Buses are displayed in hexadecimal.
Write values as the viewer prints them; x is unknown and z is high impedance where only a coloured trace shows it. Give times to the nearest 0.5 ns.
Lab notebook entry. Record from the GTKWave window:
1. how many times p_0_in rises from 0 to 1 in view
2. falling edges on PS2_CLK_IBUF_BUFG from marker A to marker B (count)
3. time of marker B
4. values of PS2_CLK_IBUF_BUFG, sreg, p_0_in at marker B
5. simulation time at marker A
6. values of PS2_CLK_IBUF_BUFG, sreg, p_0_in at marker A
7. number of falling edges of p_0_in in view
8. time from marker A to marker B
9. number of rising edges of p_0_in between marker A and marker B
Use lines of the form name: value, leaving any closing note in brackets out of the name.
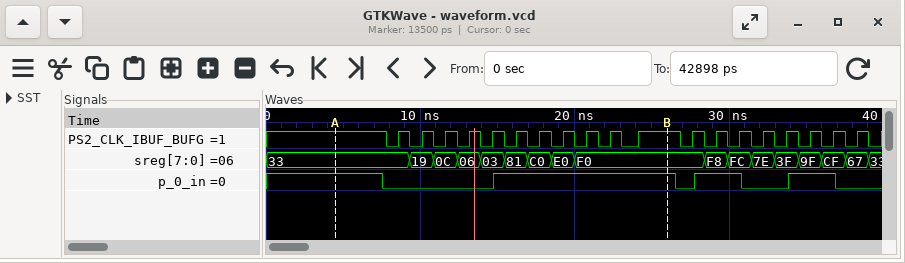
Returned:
how many times p_0_in rises from 0 to 1 in view: 3
falling edges on PS2_CLK_IBUF_BUFG from marker A to marker B: 11
time of marker B: 26 ns
values of PS2_CLK_IBUF_BUFG, sreg, p_0_in at marker B: PS2_CLK_IBUF_BUFG=1, sreg=F0, p_0_in=1
simulation time at marker A: 4.5 ns
values of PS2_CLK_IBUF_BUFG, sreg, p_0_in at marker A: PS2_CLK_IBUF_BUFG=1, sreg=33, p_0_in=1
number of falling edges of p_0_in in view: 4
time from marker A to marker B: 21.5 ns
number of rising edges of p_0_in between marker A and marker B: 1
